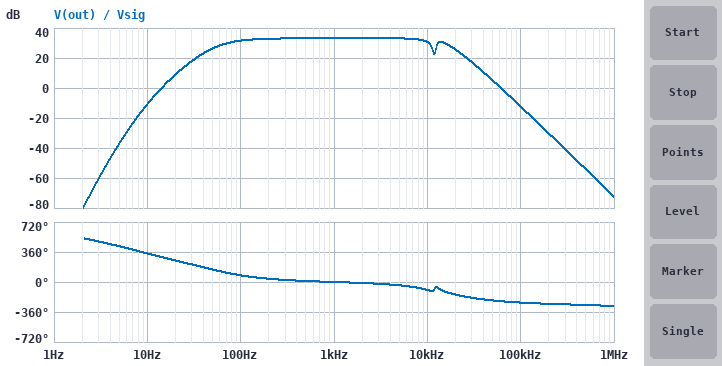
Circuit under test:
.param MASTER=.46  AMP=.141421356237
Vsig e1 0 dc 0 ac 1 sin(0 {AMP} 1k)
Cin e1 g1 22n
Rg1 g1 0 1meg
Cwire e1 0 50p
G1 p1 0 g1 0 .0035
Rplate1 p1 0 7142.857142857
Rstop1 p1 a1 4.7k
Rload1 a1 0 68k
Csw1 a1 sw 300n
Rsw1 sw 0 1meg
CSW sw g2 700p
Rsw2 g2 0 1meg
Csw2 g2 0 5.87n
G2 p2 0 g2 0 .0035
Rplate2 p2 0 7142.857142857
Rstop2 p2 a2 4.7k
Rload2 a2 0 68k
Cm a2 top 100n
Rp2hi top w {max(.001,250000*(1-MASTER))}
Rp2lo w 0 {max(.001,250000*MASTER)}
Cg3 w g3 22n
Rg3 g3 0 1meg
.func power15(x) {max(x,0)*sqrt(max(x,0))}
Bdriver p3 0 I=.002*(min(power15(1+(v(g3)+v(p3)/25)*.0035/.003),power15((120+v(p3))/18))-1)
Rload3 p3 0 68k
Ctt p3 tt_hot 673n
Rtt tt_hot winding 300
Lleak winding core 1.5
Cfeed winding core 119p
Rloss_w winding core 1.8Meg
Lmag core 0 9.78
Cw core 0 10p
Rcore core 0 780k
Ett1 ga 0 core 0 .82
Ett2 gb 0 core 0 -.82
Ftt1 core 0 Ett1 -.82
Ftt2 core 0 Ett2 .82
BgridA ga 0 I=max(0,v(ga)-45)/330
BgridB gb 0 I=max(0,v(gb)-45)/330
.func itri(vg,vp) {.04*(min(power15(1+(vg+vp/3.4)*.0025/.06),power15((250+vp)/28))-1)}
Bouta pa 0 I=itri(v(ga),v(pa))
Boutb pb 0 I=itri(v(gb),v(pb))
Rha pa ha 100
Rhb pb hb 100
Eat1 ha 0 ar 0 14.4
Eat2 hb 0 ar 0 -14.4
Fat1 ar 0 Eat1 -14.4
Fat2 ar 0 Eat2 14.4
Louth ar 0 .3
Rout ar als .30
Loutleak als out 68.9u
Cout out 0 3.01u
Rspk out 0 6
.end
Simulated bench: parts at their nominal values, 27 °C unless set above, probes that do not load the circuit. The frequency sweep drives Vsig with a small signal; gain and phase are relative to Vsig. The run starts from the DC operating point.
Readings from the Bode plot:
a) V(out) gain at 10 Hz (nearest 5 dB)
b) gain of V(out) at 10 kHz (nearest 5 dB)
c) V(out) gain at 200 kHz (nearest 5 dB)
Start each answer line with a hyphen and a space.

- -10 dB
- 30 dB
- -30 dB
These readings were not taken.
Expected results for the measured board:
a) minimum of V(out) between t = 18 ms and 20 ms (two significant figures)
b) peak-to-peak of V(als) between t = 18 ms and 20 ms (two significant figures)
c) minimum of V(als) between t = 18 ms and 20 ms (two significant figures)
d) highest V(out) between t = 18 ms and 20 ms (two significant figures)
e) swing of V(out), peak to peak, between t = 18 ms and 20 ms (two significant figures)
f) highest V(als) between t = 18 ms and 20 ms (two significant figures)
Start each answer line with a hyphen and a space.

- -6.4 V
- 13 V
- -6.4 V
- 6.4 V
- 13 V
- 6.4 V
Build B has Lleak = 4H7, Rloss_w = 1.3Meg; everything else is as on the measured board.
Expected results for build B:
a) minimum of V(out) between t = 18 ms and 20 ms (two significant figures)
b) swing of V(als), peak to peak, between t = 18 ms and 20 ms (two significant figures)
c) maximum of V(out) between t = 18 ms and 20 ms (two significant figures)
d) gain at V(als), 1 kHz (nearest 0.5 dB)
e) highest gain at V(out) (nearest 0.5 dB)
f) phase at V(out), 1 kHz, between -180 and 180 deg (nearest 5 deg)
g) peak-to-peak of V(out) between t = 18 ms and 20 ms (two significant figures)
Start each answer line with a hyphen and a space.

- -5.0 V
- 9.9 V
- 5.0 V
- 31.0 dB
- 35.0 dB
- 0 deg
- 10 V
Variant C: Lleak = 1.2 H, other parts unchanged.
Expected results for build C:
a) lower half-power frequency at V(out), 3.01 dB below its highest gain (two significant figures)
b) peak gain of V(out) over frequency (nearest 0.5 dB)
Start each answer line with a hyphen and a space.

- 77 Hz
- 33.5 dB
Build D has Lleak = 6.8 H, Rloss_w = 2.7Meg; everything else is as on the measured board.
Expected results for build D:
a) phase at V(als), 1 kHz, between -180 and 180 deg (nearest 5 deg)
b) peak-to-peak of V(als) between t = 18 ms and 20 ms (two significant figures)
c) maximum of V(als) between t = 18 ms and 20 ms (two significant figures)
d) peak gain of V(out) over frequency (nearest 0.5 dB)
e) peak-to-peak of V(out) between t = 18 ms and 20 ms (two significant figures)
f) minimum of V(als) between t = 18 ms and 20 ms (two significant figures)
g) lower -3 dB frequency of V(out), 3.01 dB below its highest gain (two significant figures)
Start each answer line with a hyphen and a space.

- 0 deg
- 8.6 V
- 4.3 V
- 37.0 dB
- 8.7 V
- -4.3 V
- 6.8 kHz
